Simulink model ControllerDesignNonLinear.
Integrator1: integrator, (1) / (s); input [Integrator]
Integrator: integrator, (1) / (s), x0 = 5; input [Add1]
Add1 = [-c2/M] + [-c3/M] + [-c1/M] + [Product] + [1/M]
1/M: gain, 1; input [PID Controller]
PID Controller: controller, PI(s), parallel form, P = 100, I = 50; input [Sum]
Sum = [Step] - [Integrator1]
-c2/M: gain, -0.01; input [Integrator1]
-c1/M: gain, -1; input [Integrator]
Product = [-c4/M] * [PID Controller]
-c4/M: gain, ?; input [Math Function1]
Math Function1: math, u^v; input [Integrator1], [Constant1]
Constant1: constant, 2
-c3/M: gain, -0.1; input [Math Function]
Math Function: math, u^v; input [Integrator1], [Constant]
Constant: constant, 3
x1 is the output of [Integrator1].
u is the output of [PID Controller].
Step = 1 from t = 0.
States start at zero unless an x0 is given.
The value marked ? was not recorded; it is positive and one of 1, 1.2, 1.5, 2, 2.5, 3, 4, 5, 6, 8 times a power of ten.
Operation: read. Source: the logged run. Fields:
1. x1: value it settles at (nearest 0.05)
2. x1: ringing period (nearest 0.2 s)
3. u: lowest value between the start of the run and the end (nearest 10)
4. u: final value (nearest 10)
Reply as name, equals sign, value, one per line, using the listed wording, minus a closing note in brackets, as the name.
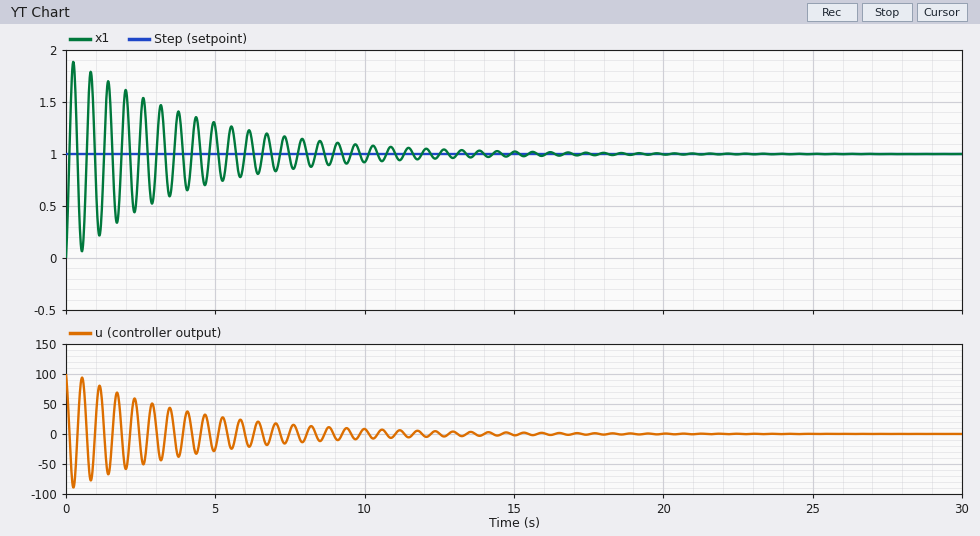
x1: value it settles at = 1.00
x1: ringing period = 0.6 s
u: lowest value between the start of the run and the end = -90
u: final value = 0
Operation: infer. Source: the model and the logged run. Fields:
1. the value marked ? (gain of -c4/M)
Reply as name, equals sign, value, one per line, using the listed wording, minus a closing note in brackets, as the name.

the value marked ? = 0.12
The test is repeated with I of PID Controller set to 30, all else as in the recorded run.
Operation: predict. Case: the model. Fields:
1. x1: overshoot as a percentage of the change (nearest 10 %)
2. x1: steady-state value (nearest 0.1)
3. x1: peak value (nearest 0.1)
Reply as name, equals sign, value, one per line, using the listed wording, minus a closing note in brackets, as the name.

x1: overshoot as a percentage of the change = 90 %
x1: steady-state value = 1.0
x1: peak value = 1.9
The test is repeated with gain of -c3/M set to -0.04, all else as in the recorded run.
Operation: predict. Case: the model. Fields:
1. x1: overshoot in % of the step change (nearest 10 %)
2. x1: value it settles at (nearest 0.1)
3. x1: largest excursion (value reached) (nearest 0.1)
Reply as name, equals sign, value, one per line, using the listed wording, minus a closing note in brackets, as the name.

x1: overshoot in % of the step change = 90 %
x1: value it settles at = 1.0
x1: largest excursion (value reached) = 1.9
